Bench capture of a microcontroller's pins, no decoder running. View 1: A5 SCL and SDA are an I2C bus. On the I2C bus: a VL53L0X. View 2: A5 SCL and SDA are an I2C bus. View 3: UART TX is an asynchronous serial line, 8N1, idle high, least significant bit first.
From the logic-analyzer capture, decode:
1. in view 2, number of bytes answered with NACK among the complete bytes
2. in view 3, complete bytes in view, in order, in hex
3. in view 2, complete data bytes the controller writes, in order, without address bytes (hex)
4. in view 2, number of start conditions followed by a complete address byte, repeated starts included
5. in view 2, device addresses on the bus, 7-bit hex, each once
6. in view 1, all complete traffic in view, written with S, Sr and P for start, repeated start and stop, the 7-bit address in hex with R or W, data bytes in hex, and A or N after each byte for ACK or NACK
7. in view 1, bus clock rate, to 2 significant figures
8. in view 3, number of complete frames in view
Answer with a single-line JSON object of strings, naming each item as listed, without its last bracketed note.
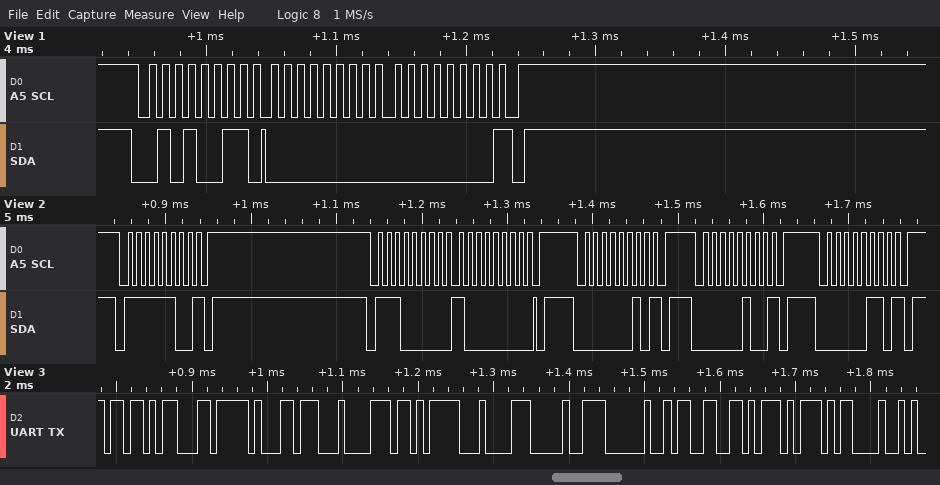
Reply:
{"in view 2, number of bytes answered with NACK among the complete bytes": "4", "in view 3, complete bytes in view, in order, in hex": "5B EC B1 84 EB 84 90 20 33 5D 0D", "in view 2, complete data bytes the controller writes, in order, without address bytes": "80", "in view 2, number of start conditions followed by a complete address byte, repeated starts included": "5", "in view 2, device addresses on the bus, 7-bit hex, each once": "0x7E 0x70 0x01 0x02 0x03", "in view 1, all complete traffic in view, written with S, Sr and P for start, repeated start and stop, the 7-bit address in hex with R or W, data bytes in hex, and A or N after each byte for ACK or NACK": "S 29R A 00 A 00 N P", "in view 1, bus clock rate, to 2 significant figures": "100 kHz", "in view 3, number of complete frames in view": "11"}
